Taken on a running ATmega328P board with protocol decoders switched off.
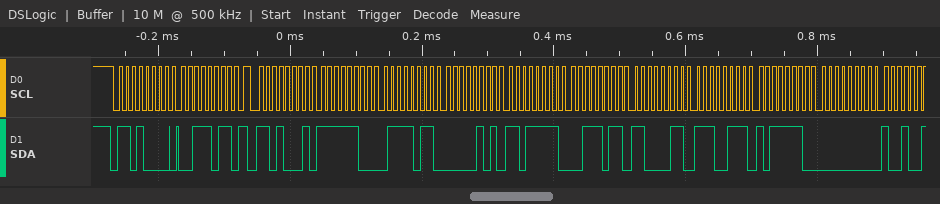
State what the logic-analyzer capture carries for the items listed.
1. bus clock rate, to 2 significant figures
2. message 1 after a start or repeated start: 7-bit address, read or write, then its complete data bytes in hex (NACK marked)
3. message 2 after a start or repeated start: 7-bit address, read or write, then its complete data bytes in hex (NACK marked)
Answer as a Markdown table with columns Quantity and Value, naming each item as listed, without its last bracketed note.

| Quantity | Value |
|---|---|
| bus clock rate, to 2 significant figures | 100 kHz |
| message 1 after a start or repeated start: 7-bit address, read or write, then its complete data bytes in hex | 0x68 write: 3B |
| message 2 after a start or repeated start: 7-bit address, read or write, then its complete data bytes in hex | 0x68 read: FC 7B 05 DF 3B C3 E7 BE 00 |
